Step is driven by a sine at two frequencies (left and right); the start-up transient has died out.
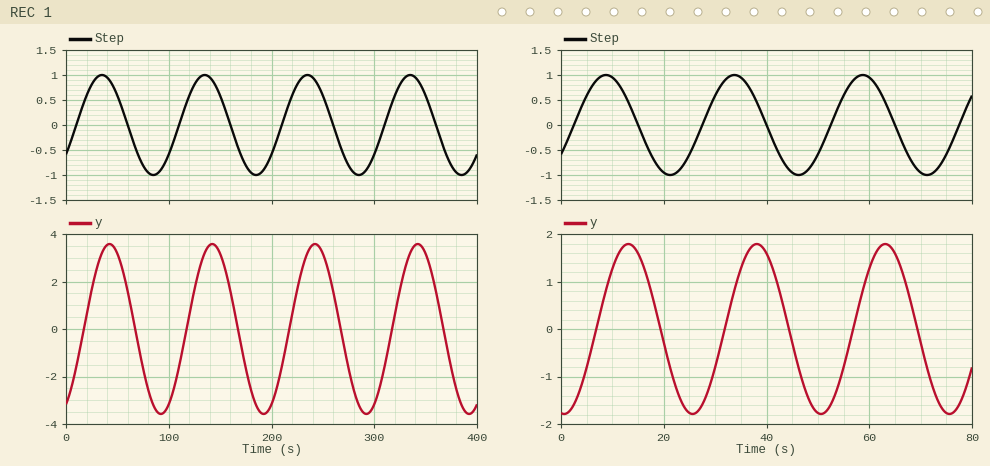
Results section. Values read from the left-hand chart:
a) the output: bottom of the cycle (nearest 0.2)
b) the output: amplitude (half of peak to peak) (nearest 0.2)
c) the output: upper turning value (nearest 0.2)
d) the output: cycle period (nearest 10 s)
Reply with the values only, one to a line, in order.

-3.6
3.6
3.6
100 s
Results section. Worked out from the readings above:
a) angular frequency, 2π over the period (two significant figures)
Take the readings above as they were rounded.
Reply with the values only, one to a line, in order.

0.063 rad/s
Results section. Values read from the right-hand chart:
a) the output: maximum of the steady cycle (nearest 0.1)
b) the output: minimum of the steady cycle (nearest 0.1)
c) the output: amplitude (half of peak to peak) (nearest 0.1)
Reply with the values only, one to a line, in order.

1.8
-1.8
1.8
